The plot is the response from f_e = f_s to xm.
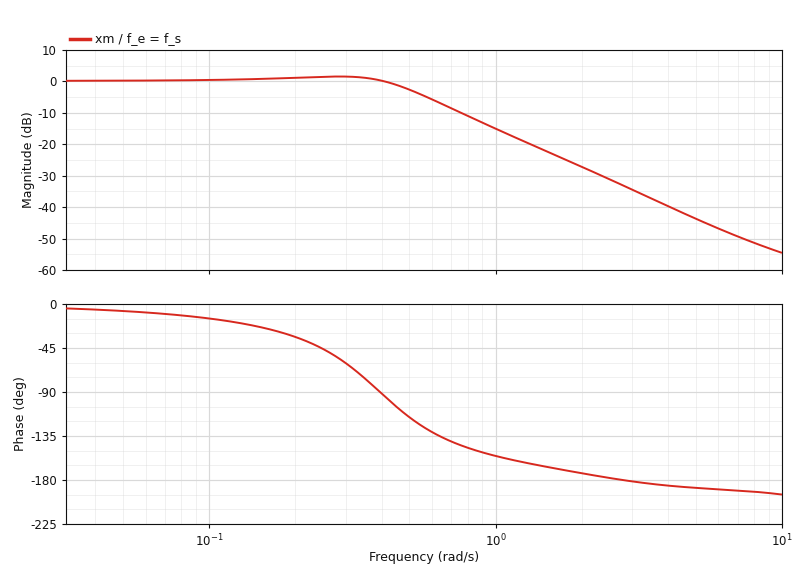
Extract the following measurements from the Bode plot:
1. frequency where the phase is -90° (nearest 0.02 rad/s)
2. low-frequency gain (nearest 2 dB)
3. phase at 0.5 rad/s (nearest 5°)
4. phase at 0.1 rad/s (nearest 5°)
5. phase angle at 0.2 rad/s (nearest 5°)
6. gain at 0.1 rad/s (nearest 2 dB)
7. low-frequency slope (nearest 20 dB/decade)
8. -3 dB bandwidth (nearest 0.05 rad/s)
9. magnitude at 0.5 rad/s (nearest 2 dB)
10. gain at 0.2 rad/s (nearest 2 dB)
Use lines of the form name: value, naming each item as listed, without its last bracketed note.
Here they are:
frequency where the phase is -90°: 0.40 rad/s
low-frequency gain: 0 dB
phase at 0.5 rad/s: -115°
phase at 0.1 rad/s: -15°
phase angle at 0.2 rad/s: -35°
gain at 0.1 rad/s: 0 dB
low-frequency slope: 0 dB/decade
-3 dB bandwidth: 0.50 rad/s
magnitude at 0.5 rad/s: -2 dB
gain at 0.2 rad/s: 2 dB
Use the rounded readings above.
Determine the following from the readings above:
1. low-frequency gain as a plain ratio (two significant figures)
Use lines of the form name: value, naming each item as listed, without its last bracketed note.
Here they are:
low-frequency gain as a plain ratio: 1.0
